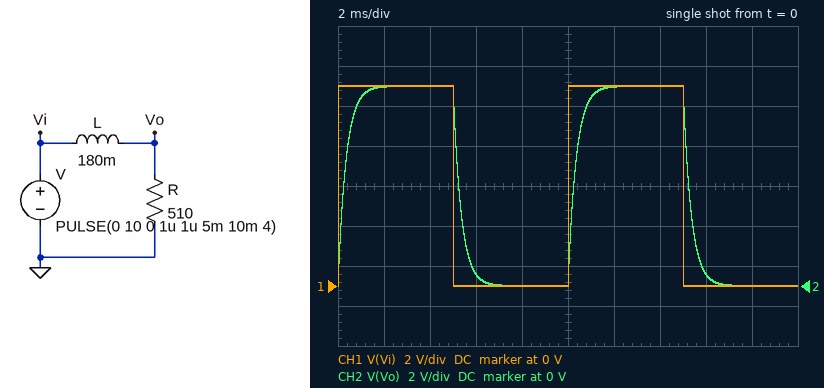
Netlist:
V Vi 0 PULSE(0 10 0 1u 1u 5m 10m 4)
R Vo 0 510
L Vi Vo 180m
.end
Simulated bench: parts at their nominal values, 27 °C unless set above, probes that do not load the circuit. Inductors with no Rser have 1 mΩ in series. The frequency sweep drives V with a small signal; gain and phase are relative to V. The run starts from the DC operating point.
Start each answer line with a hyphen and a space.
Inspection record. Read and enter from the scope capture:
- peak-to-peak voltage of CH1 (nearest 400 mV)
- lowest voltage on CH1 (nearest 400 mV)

- 10.0 V
- 0 V
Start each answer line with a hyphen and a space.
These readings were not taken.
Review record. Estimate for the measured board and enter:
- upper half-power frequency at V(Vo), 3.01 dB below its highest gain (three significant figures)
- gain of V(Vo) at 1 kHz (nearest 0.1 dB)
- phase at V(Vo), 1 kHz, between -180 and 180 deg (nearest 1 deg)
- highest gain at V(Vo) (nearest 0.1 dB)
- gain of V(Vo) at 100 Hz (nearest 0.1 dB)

- 451 Hz
- -7.7 dB
- -66 deg
- 0 dB
- -0.2 dB
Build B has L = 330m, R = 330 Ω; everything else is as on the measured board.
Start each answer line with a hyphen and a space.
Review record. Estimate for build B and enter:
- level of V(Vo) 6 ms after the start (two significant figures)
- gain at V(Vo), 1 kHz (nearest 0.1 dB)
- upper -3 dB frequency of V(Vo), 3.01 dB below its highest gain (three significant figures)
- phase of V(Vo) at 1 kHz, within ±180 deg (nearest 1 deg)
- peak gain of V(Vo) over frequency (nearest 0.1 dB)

- 3.7 V
- -16.1 dB
- 159 Hz
- -81 deg
- 0 dB
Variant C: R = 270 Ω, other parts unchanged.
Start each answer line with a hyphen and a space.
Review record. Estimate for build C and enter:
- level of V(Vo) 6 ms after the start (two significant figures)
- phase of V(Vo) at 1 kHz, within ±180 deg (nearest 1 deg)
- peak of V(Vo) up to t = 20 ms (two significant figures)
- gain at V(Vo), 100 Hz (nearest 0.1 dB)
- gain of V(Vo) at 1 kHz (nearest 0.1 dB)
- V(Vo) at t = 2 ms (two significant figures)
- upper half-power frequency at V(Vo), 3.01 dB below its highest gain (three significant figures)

- 2.2 V
- -77 deg
- 10 V
- -0.7 dB
- -12.7 dB
- 9.5 V
- 239 Hz
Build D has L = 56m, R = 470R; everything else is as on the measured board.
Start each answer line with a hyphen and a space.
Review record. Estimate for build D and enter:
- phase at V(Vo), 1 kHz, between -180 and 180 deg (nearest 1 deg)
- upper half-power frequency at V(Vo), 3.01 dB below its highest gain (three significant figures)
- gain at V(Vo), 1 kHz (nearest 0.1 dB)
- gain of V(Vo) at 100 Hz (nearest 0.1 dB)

- -37 deg
- 1.34 kHz
- -1.9 dB
- 0 dB
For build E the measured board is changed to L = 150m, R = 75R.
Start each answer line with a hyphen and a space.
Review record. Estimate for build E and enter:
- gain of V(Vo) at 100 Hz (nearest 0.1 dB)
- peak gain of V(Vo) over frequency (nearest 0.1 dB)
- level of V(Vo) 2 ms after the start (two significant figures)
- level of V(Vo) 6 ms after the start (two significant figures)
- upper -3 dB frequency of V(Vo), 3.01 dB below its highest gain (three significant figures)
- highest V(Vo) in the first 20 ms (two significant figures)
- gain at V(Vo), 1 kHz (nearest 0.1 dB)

- -4.1 dB
- 0 dB
- 6.3 V
- 5.6 V
- 79.6 Hz
- 9.2 V
- -22.0 dB
